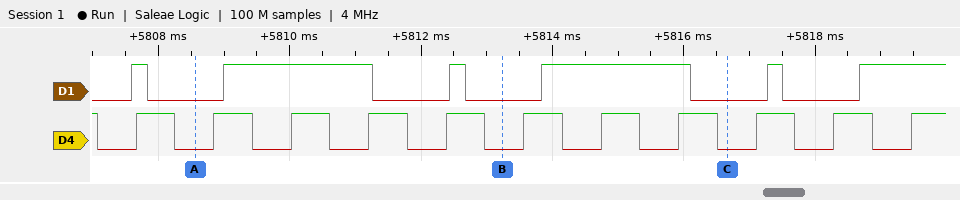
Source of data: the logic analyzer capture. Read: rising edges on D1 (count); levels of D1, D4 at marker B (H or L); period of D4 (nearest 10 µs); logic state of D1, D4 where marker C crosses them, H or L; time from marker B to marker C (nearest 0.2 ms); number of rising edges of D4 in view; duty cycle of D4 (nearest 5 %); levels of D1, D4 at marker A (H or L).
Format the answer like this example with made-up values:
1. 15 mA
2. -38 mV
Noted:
1. 6
2. D1=L, D4=L
3. 1180 µs
4. D1=L, D4=L
5. 3.4 ms
6. 11
7. 50 %
8. D1=L, D4=L
